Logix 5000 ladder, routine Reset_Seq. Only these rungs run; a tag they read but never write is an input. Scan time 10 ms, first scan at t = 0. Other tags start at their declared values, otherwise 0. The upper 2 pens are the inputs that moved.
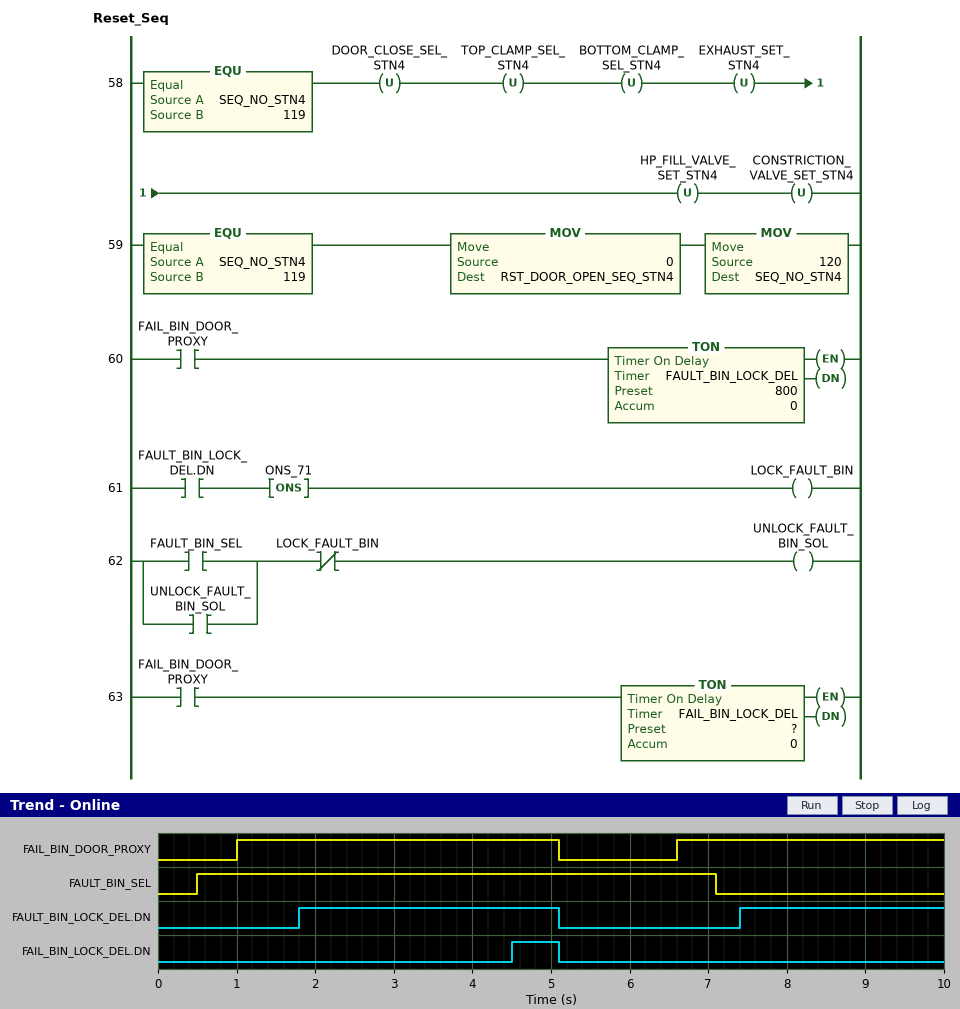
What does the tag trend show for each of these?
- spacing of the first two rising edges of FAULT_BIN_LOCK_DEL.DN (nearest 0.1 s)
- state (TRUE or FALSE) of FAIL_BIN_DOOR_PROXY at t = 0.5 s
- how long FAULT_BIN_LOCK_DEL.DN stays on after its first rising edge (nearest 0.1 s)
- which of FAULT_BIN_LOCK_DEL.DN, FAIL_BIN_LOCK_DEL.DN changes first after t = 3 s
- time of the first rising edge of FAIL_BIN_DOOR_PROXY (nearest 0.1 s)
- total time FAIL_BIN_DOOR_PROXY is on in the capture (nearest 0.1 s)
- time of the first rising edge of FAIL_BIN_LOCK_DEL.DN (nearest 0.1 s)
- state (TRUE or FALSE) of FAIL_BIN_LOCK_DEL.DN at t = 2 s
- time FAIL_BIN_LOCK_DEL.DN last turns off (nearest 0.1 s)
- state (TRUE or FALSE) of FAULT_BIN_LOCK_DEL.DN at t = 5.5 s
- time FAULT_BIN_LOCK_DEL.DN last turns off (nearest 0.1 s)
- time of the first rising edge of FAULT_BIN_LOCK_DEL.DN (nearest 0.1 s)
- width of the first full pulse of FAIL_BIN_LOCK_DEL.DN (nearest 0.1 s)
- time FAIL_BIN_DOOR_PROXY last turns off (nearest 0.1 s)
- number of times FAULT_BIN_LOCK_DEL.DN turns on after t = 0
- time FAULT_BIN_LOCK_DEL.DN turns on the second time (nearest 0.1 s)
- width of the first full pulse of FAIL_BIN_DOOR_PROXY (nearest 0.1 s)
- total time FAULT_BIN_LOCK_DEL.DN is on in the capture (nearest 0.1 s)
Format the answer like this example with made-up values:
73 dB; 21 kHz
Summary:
5.6 s; FALSE; 3.3 s; FAIL_BIN_LOCK_DEL.DN; 1.0 s; 7.5 s; 4.5 s; FALSE; 5.1 s; FALSE; 5.1 s; 1.8 s; 0.6 s; 5.1 s; 2; 7.4 s; 4.1 s; 5.9 s
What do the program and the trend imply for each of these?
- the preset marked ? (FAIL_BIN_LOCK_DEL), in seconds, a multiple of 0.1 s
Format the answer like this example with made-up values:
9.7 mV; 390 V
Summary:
3.5 s
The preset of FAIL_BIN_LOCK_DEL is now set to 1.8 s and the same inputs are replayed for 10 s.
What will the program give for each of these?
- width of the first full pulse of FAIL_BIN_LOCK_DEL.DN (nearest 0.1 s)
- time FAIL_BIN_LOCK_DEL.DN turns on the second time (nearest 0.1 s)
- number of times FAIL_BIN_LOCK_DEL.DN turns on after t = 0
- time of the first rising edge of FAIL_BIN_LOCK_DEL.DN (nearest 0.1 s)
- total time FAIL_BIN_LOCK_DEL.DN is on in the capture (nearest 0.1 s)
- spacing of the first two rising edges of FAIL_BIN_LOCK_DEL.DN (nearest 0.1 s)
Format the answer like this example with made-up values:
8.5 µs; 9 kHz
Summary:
2.3 s; 8.4 s; 2; 2.8 s; 3.9 s; 5.6 s
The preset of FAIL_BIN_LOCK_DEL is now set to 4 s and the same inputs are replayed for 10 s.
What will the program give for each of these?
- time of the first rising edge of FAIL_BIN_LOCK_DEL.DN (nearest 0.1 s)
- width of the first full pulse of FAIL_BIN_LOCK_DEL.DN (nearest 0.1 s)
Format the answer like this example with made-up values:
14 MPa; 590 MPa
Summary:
5.0 s; 0.1 s
